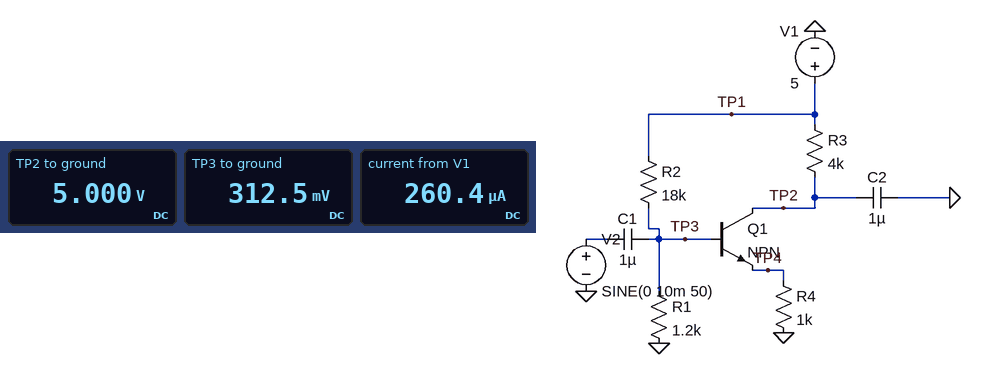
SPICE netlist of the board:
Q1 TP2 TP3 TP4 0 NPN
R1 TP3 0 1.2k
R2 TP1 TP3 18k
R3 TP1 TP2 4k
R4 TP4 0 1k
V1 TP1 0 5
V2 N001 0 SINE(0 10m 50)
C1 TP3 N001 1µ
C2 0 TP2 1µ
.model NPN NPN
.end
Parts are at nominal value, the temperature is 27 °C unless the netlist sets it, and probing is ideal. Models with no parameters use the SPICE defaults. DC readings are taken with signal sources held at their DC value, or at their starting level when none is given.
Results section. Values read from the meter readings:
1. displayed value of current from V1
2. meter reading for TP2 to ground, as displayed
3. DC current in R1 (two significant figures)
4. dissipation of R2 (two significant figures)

260.4 µA
5.000 V
260 µA
1.2 mW
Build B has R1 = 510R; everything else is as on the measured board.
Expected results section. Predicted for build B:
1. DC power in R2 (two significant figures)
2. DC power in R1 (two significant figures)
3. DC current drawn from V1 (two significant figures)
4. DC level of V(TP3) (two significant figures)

1.3 mW
37 µW
270 µA
140 mV
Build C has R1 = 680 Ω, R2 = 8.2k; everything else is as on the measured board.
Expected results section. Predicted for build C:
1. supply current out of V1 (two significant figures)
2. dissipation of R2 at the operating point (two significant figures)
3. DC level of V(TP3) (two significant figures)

560 µA
2.6 mW
380 mV
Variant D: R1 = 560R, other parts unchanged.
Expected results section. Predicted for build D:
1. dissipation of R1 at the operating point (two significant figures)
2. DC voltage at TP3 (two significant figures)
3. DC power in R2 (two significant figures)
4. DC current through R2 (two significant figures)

41 µW
150 mV
1.3 mW
270 µA
